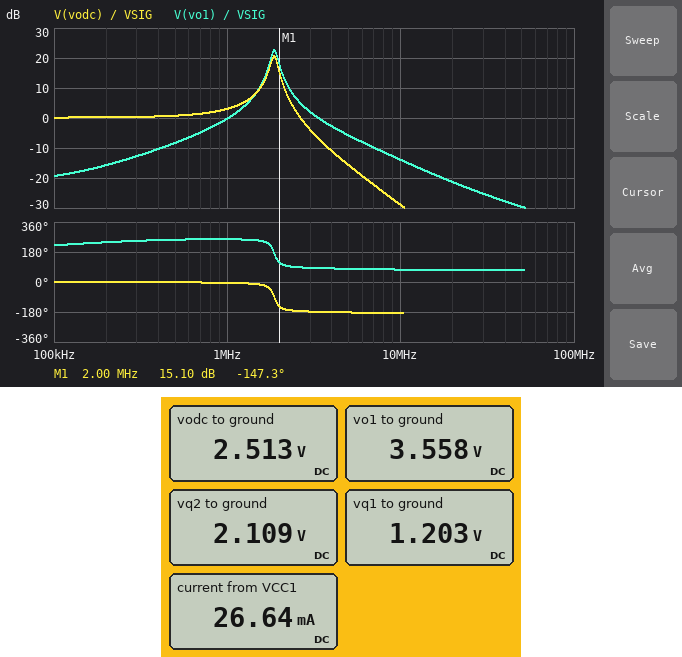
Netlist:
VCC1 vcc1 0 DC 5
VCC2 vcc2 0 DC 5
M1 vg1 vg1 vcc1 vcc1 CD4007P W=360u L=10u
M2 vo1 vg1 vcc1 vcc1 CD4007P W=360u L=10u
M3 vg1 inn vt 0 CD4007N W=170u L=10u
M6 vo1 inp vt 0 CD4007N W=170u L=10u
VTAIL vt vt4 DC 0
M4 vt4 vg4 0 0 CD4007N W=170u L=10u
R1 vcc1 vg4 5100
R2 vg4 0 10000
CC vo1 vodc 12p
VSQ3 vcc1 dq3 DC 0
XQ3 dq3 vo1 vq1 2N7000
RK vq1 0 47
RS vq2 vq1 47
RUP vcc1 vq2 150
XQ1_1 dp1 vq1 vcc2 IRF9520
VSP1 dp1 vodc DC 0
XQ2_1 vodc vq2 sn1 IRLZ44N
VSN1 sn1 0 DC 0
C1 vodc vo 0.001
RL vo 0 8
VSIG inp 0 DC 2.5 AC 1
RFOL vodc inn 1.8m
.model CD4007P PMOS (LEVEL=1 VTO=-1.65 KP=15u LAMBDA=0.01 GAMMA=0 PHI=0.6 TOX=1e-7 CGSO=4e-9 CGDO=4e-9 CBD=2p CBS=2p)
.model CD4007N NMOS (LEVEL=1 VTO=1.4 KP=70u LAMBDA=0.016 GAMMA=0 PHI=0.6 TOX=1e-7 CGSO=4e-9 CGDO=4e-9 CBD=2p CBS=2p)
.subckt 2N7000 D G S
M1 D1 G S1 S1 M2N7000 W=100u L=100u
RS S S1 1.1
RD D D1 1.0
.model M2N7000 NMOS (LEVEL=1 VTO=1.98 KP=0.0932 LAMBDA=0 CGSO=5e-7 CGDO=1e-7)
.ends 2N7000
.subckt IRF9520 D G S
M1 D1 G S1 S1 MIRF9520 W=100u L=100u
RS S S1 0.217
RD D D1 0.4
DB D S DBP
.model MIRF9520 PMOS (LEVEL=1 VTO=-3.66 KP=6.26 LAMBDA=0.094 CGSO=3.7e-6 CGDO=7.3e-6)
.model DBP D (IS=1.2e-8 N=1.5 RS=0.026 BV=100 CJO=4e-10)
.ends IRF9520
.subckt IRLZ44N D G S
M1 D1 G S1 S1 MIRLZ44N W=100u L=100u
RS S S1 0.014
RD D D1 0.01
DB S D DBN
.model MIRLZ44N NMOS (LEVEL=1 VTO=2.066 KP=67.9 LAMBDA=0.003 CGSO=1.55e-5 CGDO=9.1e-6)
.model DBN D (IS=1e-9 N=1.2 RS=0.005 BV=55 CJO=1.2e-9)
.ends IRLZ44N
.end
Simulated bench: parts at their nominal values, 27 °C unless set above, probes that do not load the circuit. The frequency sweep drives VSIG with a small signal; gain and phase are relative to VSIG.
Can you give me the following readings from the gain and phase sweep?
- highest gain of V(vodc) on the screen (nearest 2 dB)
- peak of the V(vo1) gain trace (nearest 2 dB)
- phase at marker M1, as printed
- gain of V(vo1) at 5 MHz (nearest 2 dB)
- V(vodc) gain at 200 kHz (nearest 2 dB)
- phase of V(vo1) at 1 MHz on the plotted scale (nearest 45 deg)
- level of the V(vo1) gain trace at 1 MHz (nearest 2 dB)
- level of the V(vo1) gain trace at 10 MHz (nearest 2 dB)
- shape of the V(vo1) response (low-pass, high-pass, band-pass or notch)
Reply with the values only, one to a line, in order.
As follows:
20 dB
22 dB
-147.3 deg
-6 dB
0 dB
270 deg
0 dB
-14 dB
band-pass
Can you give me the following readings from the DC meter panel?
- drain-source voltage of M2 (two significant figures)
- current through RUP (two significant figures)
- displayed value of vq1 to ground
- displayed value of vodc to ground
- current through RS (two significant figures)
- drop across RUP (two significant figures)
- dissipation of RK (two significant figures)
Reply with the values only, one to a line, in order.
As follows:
-1.4 V
19 mA
1.203 V
2.513 V
19 mA
2.9 V
31 mW
